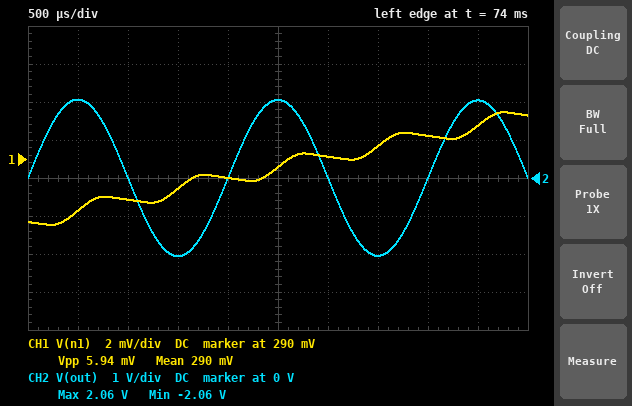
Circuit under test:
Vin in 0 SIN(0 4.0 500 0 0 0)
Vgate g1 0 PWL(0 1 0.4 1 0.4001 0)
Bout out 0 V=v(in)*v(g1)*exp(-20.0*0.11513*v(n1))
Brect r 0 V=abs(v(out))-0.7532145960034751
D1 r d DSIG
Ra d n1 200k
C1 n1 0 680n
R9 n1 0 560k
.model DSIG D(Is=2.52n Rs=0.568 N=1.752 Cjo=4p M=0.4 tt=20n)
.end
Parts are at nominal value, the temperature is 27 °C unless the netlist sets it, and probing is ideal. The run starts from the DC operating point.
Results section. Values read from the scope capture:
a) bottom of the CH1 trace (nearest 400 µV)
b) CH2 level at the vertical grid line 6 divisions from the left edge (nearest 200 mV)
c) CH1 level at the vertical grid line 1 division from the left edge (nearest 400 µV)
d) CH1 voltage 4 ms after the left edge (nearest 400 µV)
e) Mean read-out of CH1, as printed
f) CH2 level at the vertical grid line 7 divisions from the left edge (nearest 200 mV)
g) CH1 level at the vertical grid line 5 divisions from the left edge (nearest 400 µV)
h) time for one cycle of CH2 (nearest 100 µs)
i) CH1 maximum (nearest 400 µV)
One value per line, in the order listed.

286.4 mV
0 V
287.2 mV
291.2 mV
290 mV
-2.0 V
289.6 mV
2.0 ms
292.4 mV
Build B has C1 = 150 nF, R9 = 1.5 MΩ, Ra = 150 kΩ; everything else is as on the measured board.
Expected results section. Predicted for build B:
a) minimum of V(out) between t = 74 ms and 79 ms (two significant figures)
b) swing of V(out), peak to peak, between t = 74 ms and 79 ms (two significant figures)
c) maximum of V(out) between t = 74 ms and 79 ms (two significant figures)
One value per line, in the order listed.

-1.6 V
3.2 V
1.6 V
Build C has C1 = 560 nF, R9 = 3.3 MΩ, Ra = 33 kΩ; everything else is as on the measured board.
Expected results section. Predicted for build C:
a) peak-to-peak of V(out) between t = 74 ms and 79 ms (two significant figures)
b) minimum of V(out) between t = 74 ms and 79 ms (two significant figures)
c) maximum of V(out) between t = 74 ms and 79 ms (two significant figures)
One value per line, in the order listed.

3.0 V
-1.5 V
1.5 V
